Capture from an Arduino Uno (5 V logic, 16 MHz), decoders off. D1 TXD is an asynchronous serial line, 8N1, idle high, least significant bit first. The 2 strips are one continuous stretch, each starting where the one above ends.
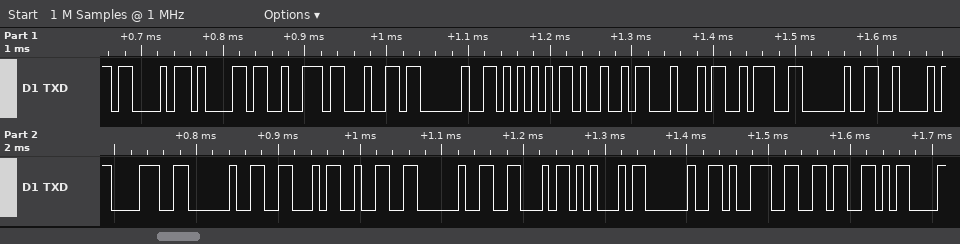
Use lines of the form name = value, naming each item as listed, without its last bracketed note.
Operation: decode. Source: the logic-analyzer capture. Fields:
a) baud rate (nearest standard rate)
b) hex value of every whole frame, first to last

baud rate = 115200 baud
hex value of every whole frame, first to last = 0x43 0x61 0x72 0x64 0x20 0x55 0x49 0x44 0x3A 0x20 0x42 0x38 0x20 0x46 0x32 0x20 0x46 0x45 0x20 0x39 0x36 0x0D
